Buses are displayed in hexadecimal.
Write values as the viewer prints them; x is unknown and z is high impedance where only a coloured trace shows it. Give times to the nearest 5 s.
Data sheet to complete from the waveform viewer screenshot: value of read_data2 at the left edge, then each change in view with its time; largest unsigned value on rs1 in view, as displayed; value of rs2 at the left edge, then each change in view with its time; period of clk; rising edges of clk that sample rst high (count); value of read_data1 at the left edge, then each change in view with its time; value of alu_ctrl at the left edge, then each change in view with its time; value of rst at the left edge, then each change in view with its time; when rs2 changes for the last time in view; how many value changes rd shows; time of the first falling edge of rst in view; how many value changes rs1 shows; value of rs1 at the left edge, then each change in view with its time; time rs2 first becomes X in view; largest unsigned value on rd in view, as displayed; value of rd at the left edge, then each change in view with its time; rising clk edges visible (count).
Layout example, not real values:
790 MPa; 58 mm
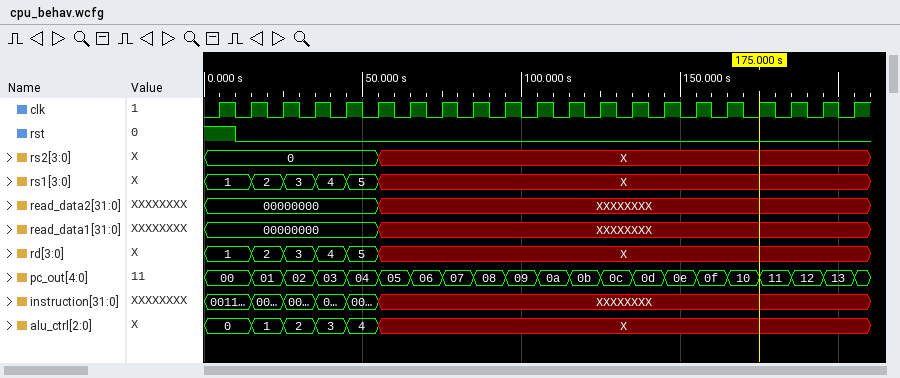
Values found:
00000000, XXXXXXXX at 55 s; 5; 0, X at 55 s; 10 s; 1; 00000000, XXXXXXXX at 55 s; 0, 1 at 15 s, 2 at 25 s, 3 at 35 s, 4 at 45 s, X at 55 s; 1, 0 at 10 s; 55 s; 5; 10 s; 5; 1, 2 at 15 s, 3 at 25 s, 4 at 35 s, 5 at 45 s, X at 55 s; 55 s; 5; 1, 2 at 15 s, 3 at 25 s, 4 at 35 s, 5 at 45 s, X at 55 s; 21
